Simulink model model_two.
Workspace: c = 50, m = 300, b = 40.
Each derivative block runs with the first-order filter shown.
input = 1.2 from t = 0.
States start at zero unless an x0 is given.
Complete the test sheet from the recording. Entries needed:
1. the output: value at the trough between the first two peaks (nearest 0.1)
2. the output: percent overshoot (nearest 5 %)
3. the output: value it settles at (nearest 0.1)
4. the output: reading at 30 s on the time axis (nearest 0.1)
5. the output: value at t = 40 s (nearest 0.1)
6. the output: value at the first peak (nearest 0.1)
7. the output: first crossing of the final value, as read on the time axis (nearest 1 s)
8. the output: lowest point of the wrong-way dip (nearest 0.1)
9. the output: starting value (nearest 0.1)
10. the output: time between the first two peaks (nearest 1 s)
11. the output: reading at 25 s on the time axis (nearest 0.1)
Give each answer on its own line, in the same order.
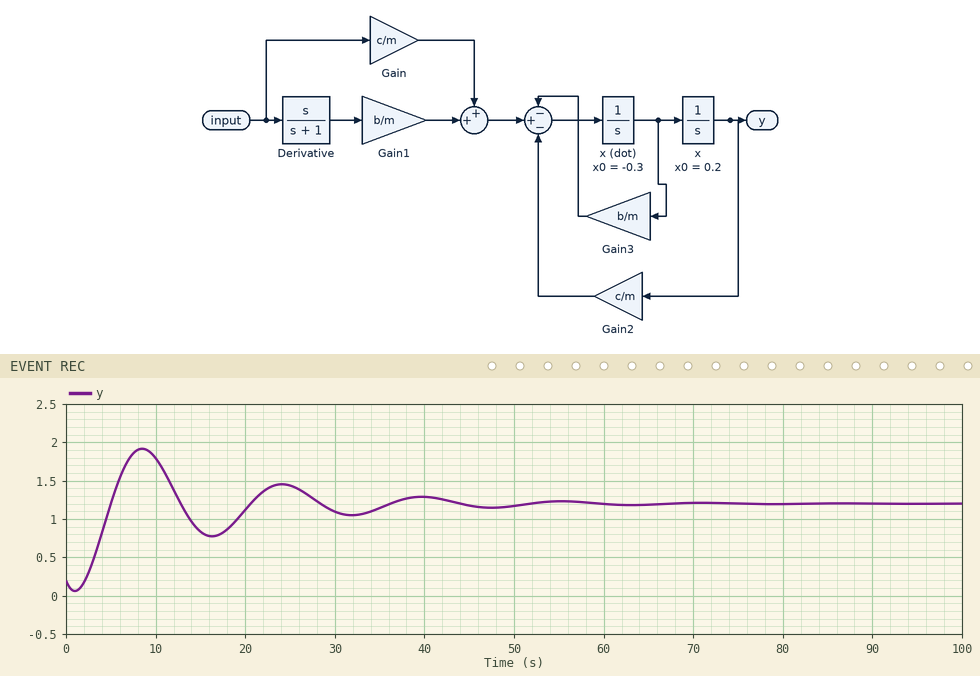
0.8
70 %
1.2
1.1
1.3
1.9
5 s
0.1
0.2
16 s
1.4
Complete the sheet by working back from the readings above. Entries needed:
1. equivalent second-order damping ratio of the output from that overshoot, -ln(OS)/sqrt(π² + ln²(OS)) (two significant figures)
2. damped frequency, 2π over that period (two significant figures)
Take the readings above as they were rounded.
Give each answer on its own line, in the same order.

0.11
0.39 rad/s
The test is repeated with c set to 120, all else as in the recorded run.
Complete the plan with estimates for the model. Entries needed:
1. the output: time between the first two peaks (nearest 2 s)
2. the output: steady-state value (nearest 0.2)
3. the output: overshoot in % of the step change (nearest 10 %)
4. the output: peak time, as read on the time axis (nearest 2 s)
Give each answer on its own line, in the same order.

10 s
1.2
80 %
6 s
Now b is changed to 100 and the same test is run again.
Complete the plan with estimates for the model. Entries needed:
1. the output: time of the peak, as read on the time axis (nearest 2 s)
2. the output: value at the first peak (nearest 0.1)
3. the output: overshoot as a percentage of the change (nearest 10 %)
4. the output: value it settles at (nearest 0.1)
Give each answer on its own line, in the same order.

8 s
1.6
40 %
1.2
